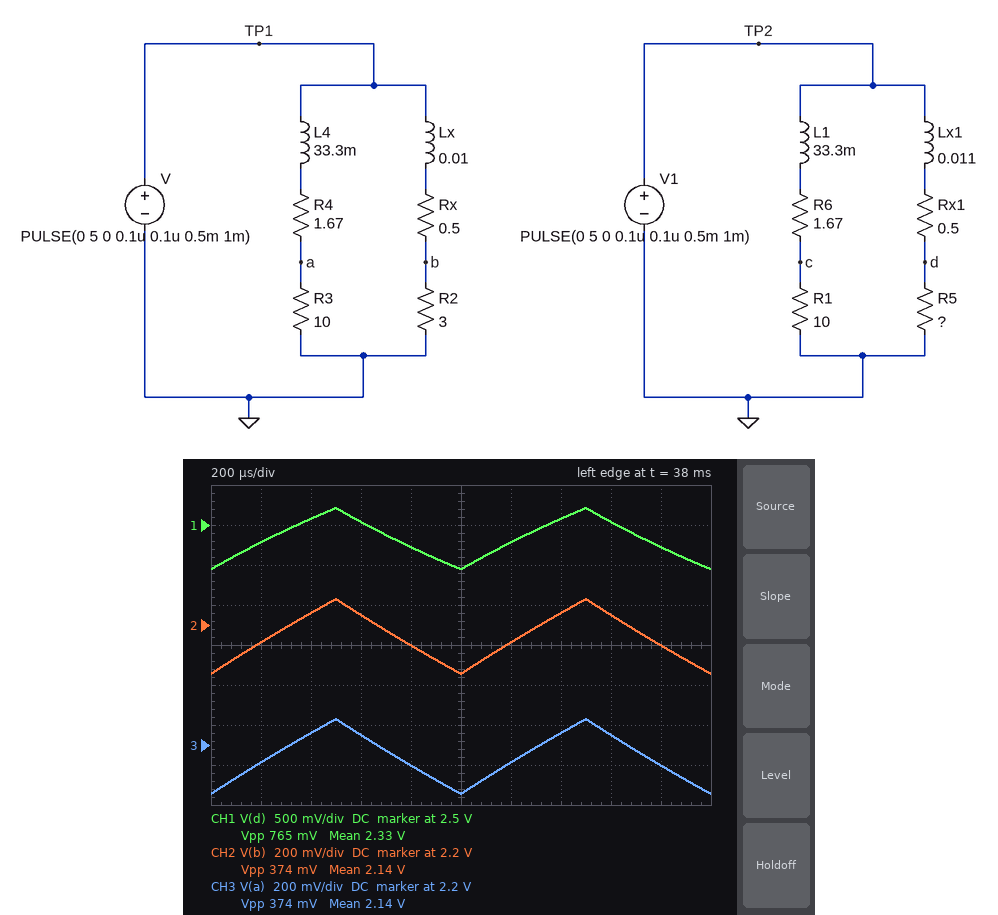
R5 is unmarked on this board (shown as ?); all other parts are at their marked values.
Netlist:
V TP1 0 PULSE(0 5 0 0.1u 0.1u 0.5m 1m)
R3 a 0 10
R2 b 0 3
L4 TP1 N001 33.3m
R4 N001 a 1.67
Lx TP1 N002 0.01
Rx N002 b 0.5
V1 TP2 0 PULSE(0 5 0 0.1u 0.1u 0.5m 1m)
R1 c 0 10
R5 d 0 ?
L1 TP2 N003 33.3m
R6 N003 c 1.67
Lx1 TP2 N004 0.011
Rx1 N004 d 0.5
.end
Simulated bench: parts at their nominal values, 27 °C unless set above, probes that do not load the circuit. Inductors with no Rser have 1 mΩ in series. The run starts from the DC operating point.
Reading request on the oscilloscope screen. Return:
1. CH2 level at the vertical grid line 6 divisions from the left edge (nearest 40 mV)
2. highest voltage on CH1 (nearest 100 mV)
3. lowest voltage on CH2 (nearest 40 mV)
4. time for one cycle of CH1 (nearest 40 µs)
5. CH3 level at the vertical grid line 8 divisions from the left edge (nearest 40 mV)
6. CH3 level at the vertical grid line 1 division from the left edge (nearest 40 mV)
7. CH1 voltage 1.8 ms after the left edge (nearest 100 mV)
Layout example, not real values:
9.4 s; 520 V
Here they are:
2.12 V; 2.7 V; 1.96 V; 1.00 ms; 2.24 V; 2.12 V; 2.2 V
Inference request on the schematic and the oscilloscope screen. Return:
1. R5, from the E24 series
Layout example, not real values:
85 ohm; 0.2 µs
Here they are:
6.8 Ω
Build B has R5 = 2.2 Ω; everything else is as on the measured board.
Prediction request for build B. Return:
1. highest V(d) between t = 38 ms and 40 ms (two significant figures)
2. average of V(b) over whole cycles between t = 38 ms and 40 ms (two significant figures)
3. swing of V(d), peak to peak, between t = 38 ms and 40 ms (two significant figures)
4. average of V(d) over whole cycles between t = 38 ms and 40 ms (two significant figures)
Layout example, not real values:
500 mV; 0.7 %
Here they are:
2.2 V; 2.1 V; 250 mV; 2.0 V
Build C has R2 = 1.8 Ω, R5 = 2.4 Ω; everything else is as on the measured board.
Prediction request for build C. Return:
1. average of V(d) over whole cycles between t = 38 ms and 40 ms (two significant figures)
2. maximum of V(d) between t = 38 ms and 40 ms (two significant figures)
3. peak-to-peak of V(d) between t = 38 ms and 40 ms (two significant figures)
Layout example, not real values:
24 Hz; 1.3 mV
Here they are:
2.1 V; 2.2 V; 270 mV
